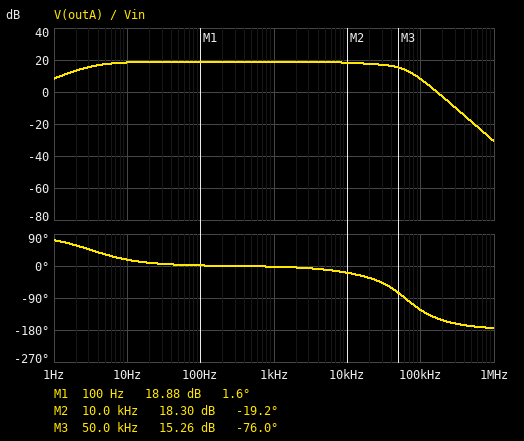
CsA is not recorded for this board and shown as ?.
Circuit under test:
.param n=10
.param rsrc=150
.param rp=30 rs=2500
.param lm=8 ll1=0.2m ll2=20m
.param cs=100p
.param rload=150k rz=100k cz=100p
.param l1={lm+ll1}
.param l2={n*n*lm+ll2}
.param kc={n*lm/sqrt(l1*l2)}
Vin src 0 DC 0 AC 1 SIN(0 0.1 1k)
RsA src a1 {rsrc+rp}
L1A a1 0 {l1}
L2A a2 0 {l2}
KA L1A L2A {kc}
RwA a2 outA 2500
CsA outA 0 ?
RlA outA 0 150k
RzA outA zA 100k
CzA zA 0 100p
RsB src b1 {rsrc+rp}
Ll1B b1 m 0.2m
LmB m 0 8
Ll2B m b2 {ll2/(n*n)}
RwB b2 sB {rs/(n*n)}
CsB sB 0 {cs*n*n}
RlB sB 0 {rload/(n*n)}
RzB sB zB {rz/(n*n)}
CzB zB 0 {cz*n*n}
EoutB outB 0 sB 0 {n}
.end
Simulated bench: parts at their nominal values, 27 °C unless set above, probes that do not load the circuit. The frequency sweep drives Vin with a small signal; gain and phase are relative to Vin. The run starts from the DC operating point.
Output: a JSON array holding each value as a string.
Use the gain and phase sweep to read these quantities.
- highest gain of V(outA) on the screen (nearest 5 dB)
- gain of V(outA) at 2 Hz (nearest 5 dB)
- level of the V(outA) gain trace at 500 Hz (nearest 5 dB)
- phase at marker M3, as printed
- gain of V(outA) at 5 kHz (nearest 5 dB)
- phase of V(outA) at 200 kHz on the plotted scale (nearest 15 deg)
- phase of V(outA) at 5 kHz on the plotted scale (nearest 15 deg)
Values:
["20 dB", "15 dB", "20 dB", "-76.0 deg", "20 dB", "-150 deg", "-15 deg"]
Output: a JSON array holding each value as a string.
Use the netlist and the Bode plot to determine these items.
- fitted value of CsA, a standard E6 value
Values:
["220 pF"]
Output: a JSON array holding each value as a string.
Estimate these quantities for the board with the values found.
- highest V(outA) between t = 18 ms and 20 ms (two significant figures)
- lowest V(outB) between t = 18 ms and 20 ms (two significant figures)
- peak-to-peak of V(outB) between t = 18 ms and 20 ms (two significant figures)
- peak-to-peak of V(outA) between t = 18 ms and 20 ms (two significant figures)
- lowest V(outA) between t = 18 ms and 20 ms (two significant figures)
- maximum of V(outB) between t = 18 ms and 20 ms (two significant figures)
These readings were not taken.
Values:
["880 mV", "-880 mV", "1.8 V", "1.8 V", "-880 mV", "880 mV"]
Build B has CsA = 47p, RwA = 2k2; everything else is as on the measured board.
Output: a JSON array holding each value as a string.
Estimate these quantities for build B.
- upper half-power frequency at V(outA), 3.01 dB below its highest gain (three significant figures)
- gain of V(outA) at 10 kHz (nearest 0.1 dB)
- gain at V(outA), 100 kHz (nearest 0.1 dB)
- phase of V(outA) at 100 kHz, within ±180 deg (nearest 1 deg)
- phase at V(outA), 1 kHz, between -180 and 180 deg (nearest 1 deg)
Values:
["151 kHz", "18.5 dB", "18.6 dB", "-62 deg", "-1 deg"]
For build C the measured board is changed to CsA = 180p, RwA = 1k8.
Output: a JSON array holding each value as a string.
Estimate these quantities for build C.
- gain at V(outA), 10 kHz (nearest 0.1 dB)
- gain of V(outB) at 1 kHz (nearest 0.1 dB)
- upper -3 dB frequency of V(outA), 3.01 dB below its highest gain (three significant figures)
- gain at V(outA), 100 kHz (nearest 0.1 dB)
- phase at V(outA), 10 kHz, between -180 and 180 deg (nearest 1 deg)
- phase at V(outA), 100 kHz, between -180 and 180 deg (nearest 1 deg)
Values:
["18.4 dB", "18.9 dB", "57.3 kHz", "10.2 dB", "-16 deg", "-120 deg"]
